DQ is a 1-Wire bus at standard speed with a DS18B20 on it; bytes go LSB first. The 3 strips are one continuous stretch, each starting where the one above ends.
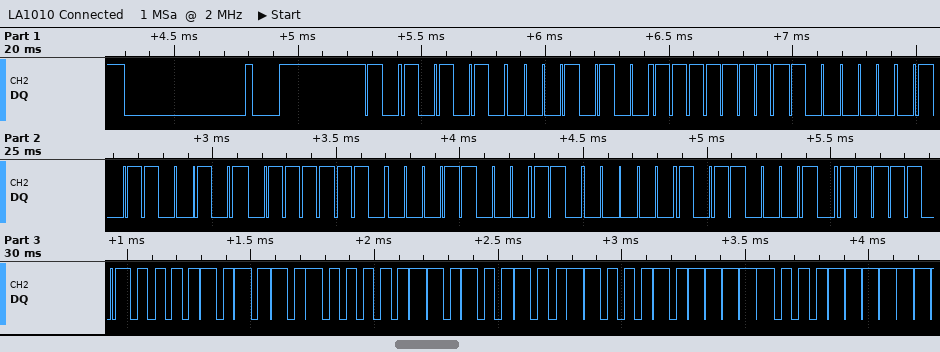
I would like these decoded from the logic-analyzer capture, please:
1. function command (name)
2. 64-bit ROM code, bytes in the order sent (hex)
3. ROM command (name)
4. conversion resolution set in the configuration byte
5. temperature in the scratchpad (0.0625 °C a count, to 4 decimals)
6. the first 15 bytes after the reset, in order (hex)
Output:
Read Scratchpad
28 FF 81 A6 7E 18 03 8D
Match ROM
9 bits
85.0000 °C
55 28 FF 81 A6 7E 18 03 8D BE 50 05 4B 46 1F
